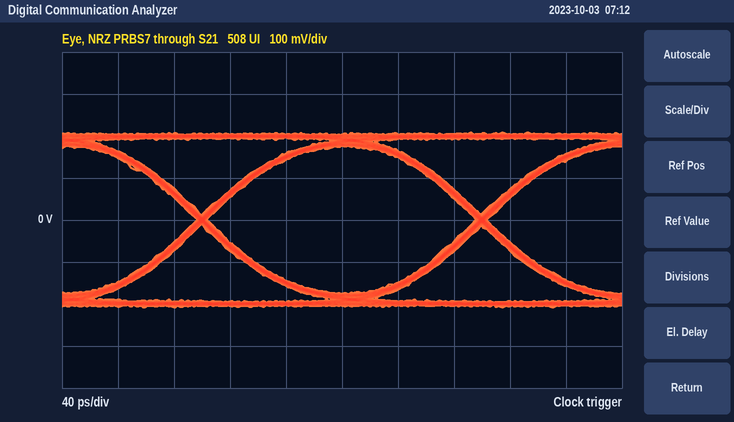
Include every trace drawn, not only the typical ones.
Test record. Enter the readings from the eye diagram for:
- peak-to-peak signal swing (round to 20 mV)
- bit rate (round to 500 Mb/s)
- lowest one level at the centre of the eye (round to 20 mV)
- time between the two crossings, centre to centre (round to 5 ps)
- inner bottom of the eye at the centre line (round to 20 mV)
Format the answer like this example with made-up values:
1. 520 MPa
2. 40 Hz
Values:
1. 420 mV
2. 5.0 Gb/s
3. 180 mV
4. 200 ps
5. -180 mV
